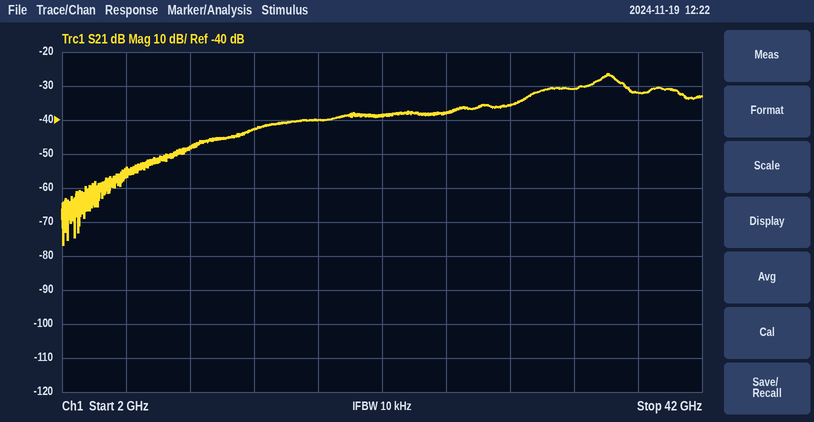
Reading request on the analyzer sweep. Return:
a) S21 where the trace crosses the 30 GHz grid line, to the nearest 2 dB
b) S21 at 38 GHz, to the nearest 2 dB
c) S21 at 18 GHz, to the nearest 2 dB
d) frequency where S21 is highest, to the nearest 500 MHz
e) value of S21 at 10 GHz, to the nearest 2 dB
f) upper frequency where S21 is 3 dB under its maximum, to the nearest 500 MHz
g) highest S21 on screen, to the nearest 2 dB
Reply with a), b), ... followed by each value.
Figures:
a) -36 dB
b) -32 dB
c) -40 dB
d) 36.0 GHz
e) -48 dB
f) 37.0 GHz
g) -26 dB
